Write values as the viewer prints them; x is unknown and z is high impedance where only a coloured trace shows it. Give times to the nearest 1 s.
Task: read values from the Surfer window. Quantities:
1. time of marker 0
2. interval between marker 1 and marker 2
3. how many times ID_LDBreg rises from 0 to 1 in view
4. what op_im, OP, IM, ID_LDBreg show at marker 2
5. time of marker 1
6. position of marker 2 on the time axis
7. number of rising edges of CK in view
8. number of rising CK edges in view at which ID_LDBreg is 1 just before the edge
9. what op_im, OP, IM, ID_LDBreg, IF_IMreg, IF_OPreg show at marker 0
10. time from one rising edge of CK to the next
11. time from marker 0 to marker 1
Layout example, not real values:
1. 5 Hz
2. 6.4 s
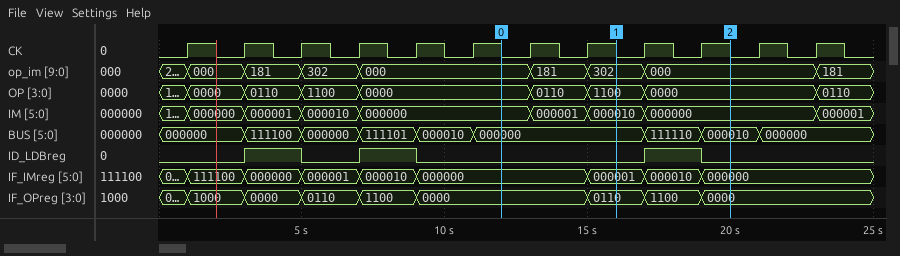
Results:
1. 12 s
2. 4 s
3. 3
4. op_im=000, OP=0000, IM=000000, ID_LDBreg=0
5. 16 s
6. 20 s
7. 12
8. 3
9. op_im=000, OP=0000, IM=000000, ID_LDBreg=0, IF_IMreg=000000, IF_OPreg=0000
10. 2 s
11. 4 s
